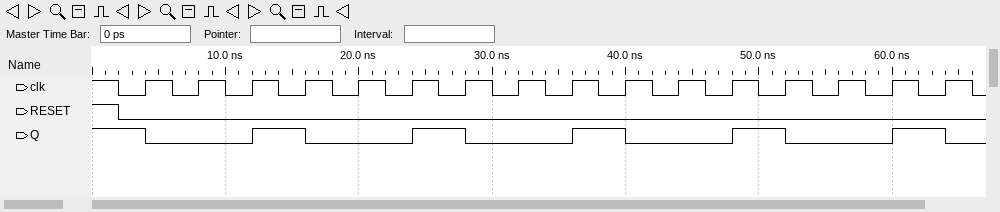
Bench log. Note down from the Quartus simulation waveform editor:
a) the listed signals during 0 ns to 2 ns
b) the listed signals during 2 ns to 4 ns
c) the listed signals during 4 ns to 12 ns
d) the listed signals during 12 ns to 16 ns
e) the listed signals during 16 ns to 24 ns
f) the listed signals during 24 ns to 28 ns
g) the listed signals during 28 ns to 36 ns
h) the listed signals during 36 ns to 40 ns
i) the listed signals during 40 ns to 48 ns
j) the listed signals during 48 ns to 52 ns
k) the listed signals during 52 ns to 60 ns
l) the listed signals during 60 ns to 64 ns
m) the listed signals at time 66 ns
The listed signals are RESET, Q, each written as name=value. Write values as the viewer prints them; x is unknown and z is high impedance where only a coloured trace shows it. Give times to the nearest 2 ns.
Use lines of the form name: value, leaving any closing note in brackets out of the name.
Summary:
the listed signals during 0 ns to 2 ns: RESET=1, Q=1
the listed signals during 2 ns to 4 ns: RESET=0, Q=1
the listed signals during 4 ns to 12 ns: RESET=0, Q=0
the listed signals during 12 ns to 16 ns: RESET=0, Q=1
the listed signals during 16 ns to 24 ns: RESET=0, Q=0
the listed signals during 24 ns to 28 ns: RESET=0, Q=1
the listed signals during 28 ns to 36 ns: RESET=0, Q=0
the listed signals during 36 ns to 40 ns: RESET=0, Q=1
the listed signals during 40 ns to 48 ns: RESET=0, Q=0
the listed signals during 48 ns to 52 ns: RESET=0, Q=1
the listed signals during 52 ns to 60 ns: RESET=0, Q=0
the listed signals during 60 ns to 64 ns: RESET=0, Q=1
the listed signals at time 66 ns: RESET=0, Q=0
